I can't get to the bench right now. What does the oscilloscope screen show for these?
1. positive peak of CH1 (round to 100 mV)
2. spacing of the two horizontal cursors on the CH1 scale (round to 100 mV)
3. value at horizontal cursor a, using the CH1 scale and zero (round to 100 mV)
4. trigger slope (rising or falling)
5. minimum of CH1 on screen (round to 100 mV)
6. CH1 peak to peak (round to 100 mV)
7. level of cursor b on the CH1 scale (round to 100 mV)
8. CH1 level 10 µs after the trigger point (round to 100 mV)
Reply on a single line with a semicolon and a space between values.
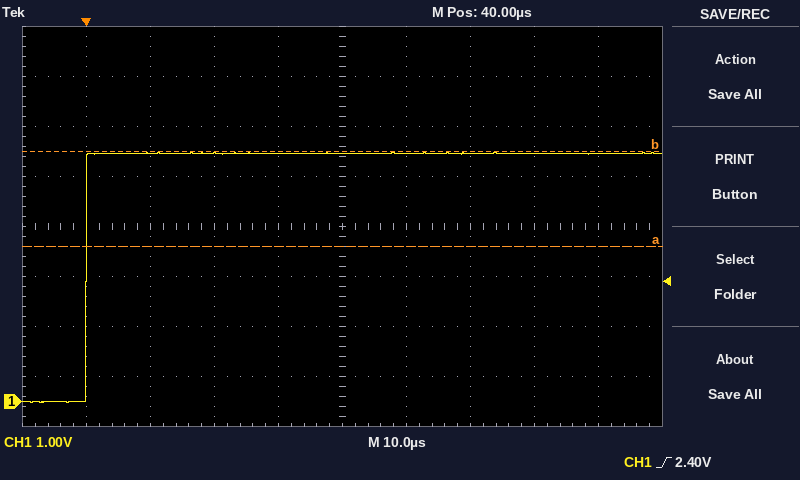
5.0 V; 1.9 V; 3.1 V; rising; 0.0 V; 5.0 V; 5.0 V; 5.0 V
